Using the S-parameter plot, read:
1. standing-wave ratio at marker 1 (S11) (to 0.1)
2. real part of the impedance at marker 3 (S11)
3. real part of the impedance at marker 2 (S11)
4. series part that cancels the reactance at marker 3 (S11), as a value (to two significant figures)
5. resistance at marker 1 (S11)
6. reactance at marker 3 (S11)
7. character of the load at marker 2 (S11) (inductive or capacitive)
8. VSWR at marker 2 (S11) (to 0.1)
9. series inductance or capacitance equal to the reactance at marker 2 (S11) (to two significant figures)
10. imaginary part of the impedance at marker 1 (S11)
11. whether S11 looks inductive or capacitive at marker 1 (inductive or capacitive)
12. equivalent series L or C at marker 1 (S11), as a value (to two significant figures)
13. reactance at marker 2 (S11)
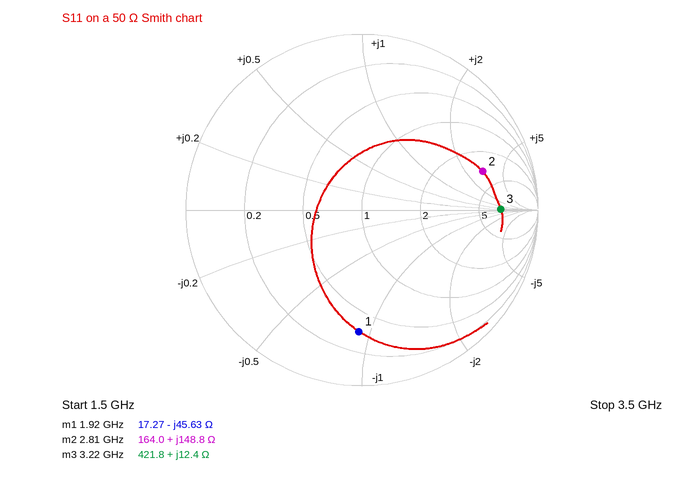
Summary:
5.5
421.8 Ω
164.0 Ω
4.0 pF
17.27 Ω
+12.4 Ω
inductive
6.1
8.4 nH
-45.63 Ω
capacitive
1.8 pF
+148.8 Ω
